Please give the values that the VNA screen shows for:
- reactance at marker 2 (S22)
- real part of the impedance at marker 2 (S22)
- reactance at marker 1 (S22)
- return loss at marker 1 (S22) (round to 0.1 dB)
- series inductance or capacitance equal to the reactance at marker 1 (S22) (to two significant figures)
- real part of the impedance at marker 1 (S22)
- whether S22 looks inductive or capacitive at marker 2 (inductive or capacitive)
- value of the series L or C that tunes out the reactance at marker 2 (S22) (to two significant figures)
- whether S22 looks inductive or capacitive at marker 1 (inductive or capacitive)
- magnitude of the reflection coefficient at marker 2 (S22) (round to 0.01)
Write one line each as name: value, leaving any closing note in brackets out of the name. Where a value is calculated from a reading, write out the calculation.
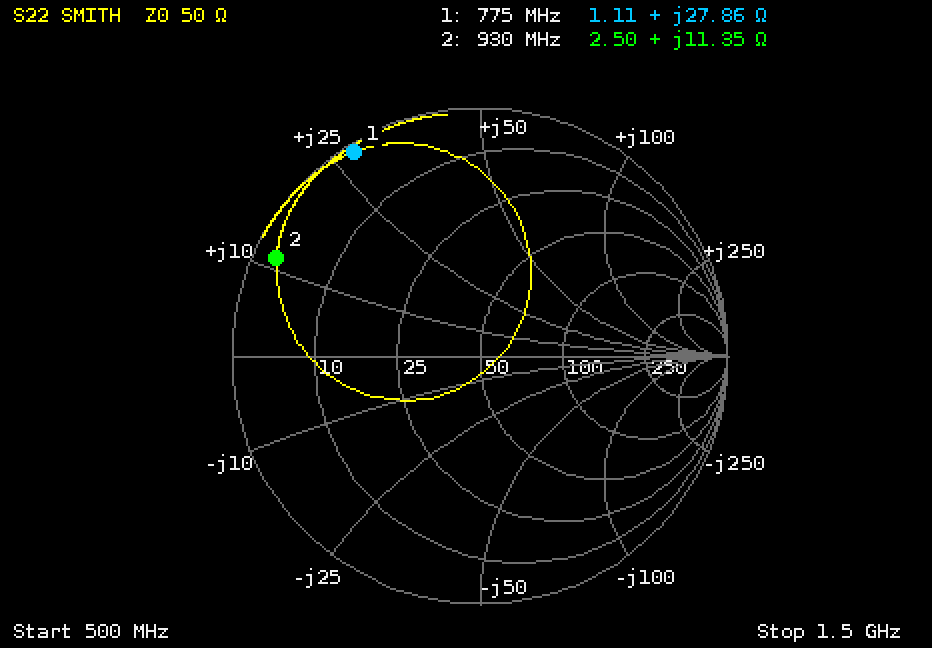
reactance at marker 2: +11.35 Ω
real part of the impedance at marker 2: 2.50 Ω
reactance at marker 1: +27.86 Ω
return loss at marker 1 (S22): 0.3 dB
series inductance or capacitance equal to the reactance at marker 1 (S22): L = 27.86 Ω/(2π × 775 MHz) ≈ 5.7 nH
real part of the impedance at marker 1: 1.11 Ω
whether S22 looks inductive or capacitive at marker 2: inductive
value of the series L or C that tunes out the reactance at marker 2 (S22): C = 1/(2π × 930 MHz × 11.35 Ω) ≈ 15 pF
whether S22 looks inductive or capacitive at marker 1: inductive
magnitude of the reflection coefficient at marker 2 (S22): 0.91
